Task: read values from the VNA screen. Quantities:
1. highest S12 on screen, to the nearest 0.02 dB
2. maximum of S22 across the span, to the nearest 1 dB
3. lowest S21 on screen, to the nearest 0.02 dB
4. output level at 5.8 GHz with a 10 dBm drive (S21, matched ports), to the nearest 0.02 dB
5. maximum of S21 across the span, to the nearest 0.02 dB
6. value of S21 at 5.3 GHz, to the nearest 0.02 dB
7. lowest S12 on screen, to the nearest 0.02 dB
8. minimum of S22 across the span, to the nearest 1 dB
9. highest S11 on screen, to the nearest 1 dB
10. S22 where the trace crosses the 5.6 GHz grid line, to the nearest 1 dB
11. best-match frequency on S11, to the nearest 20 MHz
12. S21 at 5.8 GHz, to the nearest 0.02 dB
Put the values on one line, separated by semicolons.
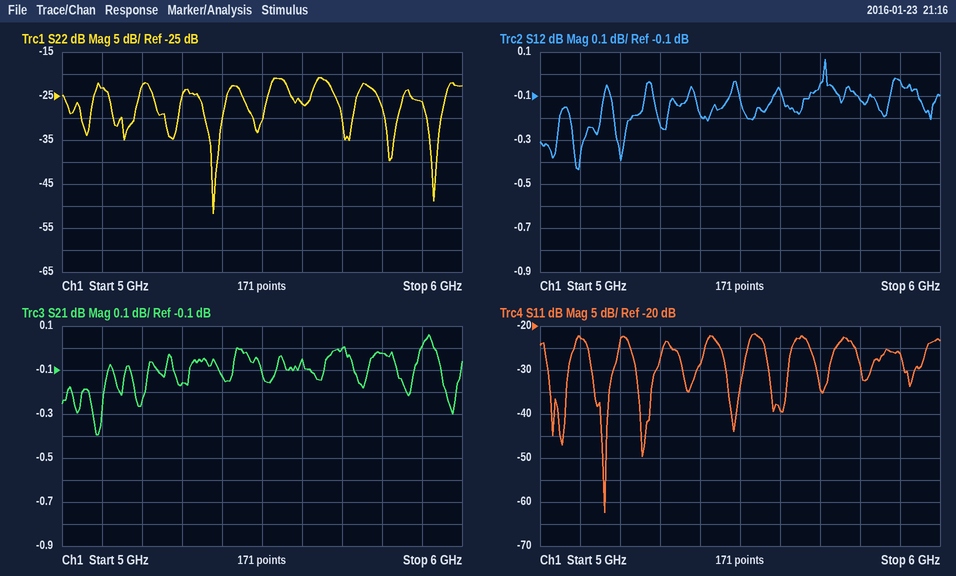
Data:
0.06 dB; -21 dB; -0.40 dB; 9.98 dBm; 0.06 dB; -0.16 dB; -0.44 dB; -52 dB; -22 dB; -27 dB; 5.16 GHz; -0.02 dB
